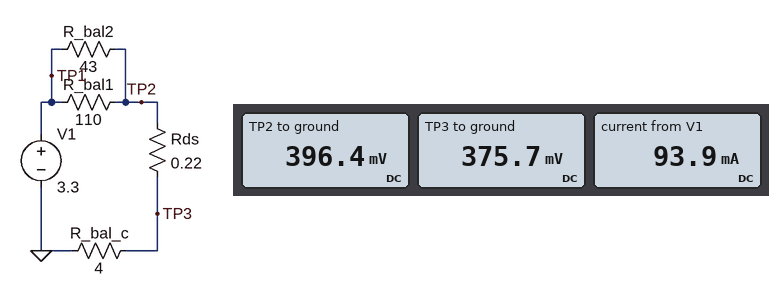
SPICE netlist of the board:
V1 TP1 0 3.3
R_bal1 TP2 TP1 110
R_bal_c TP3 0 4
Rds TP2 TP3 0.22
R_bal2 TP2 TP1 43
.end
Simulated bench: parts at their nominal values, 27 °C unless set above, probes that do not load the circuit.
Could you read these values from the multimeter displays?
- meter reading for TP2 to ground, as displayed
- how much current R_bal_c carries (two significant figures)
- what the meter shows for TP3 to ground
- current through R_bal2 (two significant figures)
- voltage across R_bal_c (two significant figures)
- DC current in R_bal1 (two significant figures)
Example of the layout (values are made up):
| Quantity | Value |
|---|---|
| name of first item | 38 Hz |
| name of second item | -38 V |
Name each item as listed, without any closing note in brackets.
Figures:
| Quantity | Value |
|---|---|
| meter reading for TP2 to ground, as displayed | 396.4 mV |
| how much current R_bal_c carries | 94 mA |
| what the meter shows for TP3 to ground | 375.7 mV |
| current through R_bal2 | 68 mA |
| voltage across R_bal_c | 380 mV |
| DC current in R_bal1 | 26 mA |
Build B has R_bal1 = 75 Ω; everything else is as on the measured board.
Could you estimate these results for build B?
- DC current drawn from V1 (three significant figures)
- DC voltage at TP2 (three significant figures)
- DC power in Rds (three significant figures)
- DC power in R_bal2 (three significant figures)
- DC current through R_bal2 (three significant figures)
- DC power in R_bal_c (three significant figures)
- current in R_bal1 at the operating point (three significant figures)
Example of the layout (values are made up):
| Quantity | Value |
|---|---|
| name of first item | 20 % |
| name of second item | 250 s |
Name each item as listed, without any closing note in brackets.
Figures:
| Quantity | Value |
|---|---|
| DC current drawn from V1 | 105 mA |
| DC voltage at TP2 | 441 mV |
| DC power in Rds | 2.41 mW |
| DC power in R_bal2 | 190 mW |
| DC current through R_bal2 | 66.5 mA |
| DC power in R_bal_c | 43.8 mW |
| current in R_bal1 at the operating point | 38.1 mA |
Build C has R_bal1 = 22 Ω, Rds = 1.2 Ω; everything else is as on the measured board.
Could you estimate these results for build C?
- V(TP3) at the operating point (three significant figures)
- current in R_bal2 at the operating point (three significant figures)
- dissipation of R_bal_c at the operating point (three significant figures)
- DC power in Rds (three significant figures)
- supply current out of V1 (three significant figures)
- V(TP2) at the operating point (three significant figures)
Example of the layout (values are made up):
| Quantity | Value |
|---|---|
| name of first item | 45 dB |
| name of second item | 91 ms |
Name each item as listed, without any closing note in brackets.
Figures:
| Quantity | Value |
|---|---|
| V(TP3) at the operating point | 668 mV |
| current in R_bal2 at the operating point | 56.5 mA |
| dissipation of R_bal_c at the operating point | 112 mW |
| DC power in Rds | 33.5 mW |
| supply current out of V1 | 167 mA |
| V(TP2) at the operating point | 869 mV |
